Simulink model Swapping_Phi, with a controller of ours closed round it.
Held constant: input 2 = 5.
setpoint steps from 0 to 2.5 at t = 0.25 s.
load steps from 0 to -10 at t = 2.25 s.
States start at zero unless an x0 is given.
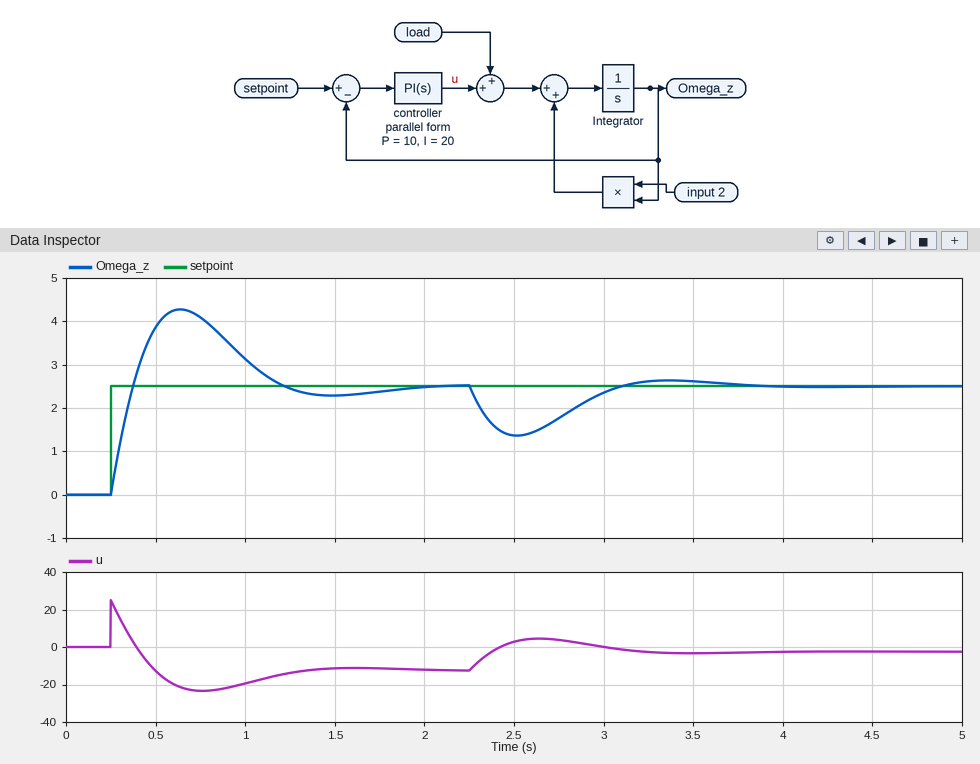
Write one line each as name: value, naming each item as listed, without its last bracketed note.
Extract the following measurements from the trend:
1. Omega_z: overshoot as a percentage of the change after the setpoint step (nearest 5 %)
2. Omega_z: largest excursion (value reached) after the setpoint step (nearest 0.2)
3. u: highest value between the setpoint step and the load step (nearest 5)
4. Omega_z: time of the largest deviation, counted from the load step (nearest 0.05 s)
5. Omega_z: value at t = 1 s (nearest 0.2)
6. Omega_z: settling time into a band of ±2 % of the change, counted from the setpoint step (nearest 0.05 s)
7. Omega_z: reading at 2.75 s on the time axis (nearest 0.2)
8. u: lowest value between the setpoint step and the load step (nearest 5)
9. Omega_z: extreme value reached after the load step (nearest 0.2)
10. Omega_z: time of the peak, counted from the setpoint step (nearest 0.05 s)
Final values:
Omega_z: overshoot as a percentage of the change after the setpoint step: 70 %
Omega_z: largest excursion (value reached) after the setpoint step: 4.2
u: highest value between the setpoint step and the load step: 25
Omega_z: time of the largest deviation, counted from the load step: 0.25 s
Omega_z: value at t = 1 s: 3.2
Omega_z: settling time into a band of ±2 % of the change, counted from the setpoint step: 1.65 s
Omega_z: reading at 2.75 s on the time axis: 1.8
u: lowest value between the setpoint step and the load step: -25
Omega_z: extreme value reached after the load step: 1.4
Omega_z: time of the peak, counted from the setpoint step: 0.40 s
